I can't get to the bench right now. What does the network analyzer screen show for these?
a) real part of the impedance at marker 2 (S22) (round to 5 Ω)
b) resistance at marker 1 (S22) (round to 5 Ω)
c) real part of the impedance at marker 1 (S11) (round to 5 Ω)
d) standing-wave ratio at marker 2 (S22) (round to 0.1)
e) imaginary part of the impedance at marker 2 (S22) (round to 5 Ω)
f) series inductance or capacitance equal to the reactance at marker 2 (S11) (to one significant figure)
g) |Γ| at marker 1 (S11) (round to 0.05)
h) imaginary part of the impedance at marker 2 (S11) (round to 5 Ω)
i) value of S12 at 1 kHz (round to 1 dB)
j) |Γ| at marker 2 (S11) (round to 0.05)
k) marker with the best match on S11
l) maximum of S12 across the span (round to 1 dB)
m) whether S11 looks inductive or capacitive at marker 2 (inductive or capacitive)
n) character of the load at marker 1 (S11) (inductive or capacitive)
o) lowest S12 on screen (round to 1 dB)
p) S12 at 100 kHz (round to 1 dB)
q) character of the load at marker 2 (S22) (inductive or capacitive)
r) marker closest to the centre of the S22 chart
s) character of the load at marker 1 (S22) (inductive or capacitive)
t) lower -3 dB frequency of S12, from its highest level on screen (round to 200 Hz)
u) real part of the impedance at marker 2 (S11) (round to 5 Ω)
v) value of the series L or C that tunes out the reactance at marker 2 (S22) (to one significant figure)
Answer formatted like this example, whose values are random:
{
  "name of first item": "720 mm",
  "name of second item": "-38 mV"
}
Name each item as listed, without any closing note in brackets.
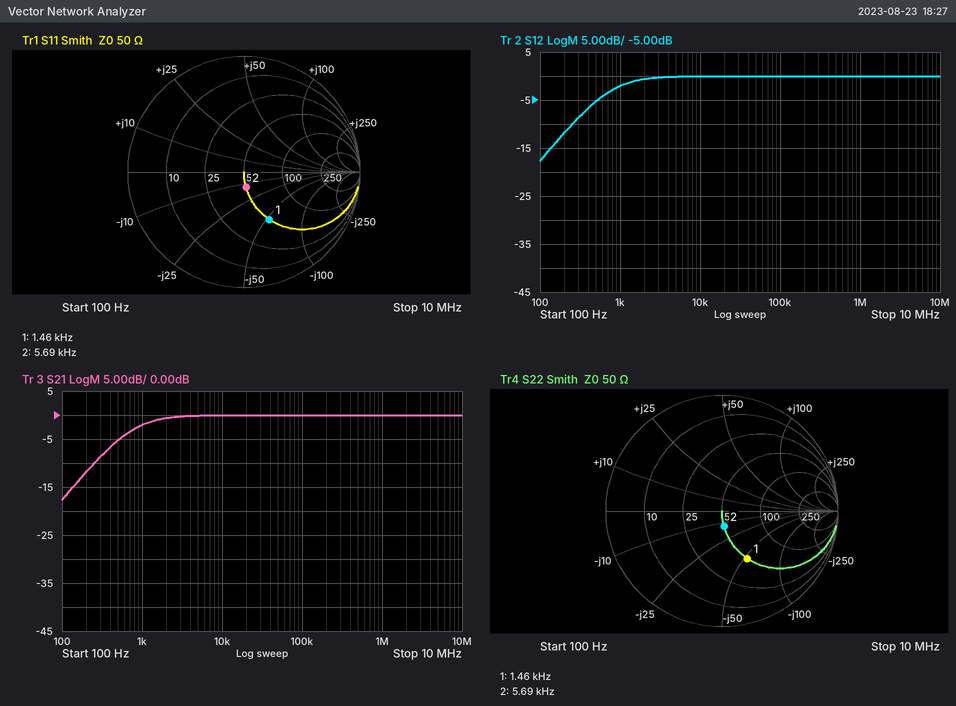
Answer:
{
  "real part of the impedance at marker 2 (S22)": "50 Ω",
  "resistance at marker 1 (S22)": "50 Ω",
  "real part of the impedance at marker 1 (S11)": "50 Ω",
  "standing-wave ratio at marker 2 (S22)": "1.3",
  "imaginary part of the impedance at marker 2 (S22)": "-15 Ω",
  "series inductance or capacitance equal to the reactance at marker 2 (S11)": "2 µF",
  "|Γ| at marker 1 (S11)": "0.45",
  "imaginary part of the impedance at marker 2 (S11)": "-15 Ω",
  "value of S12 at 1 kHz": "-2 dB",
  "|Γ| at marker 2 (S11)": "0.15",
  "marker with the best match on S11": "marker 2",
  "maximum of S12 across the span": "0 dB",
  "whether S11 looks inductive or capacitive at marker 2": "capacitive",
  "character of the load at marker 1 (S11)": "capacitive",
  "lowest S12 on screen": "-18 dB",
  "S12 at 100 kHz": "0 dB",
  "character of the load at marker 2 (S22)": "capacitive",
  "marker closest to the centre of the S22 chart": "marker 2",
  "character of the load at marker 1 (S22)": "capacitive",
  "lower -3 dB frequency of S12, from its highest level on screen": "800 Hz",
  "real part of the impedance at marker 2 (S11)": "50 Ω",
  "value of the series L or C that tunes out the reactance at marker 2 (S22)": "400 µH"
}
